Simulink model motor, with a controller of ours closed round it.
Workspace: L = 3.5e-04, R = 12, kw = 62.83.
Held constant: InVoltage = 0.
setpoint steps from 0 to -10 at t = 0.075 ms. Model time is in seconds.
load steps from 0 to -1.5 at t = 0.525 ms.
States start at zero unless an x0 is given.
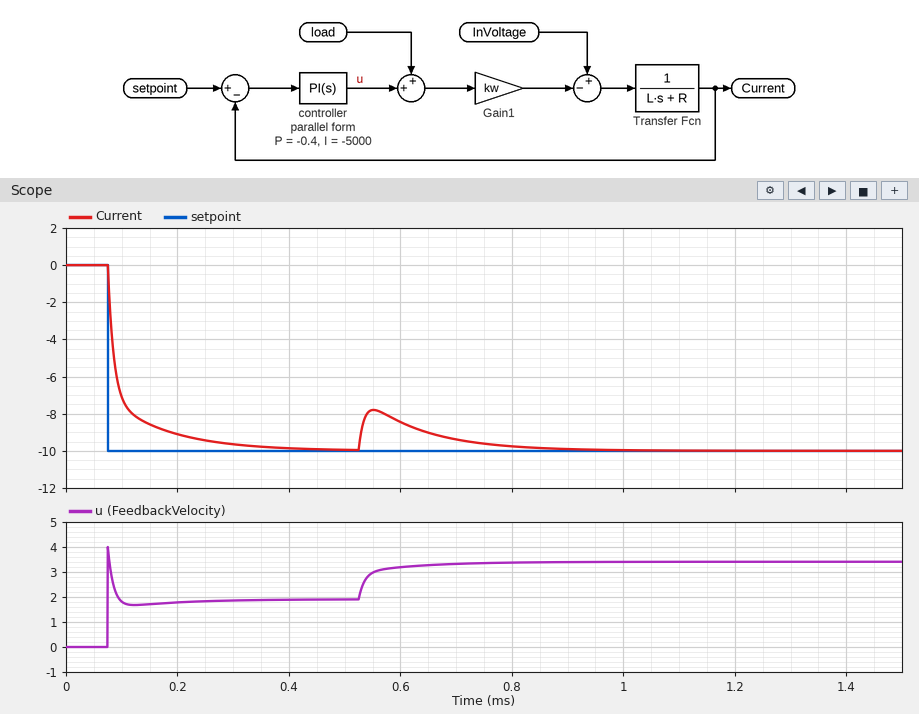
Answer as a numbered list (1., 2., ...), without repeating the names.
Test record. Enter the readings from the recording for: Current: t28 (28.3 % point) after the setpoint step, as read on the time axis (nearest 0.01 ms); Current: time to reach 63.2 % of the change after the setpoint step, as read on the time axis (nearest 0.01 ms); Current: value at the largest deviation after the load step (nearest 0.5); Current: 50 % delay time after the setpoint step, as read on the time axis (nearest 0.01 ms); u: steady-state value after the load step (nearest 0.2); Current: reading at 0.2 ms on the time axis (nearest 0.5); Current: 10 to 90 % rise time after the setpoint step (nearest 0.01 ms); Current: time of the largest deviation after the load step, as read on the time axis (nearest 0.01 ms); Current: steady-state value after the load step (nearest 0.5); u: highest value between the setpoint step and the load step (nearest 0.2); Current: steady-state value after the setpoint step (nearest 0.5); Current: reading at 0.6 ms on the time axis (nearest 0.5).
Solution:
1. 0.08 ms
2. 0.09 ms
3. -8.0
4. 0.09 ms
5. 3.4
6. -9.0
7. 0.11 ms
8. 0.55 ms
9. -10.0
10. 4.0
11. -10.0
12. -8.5
